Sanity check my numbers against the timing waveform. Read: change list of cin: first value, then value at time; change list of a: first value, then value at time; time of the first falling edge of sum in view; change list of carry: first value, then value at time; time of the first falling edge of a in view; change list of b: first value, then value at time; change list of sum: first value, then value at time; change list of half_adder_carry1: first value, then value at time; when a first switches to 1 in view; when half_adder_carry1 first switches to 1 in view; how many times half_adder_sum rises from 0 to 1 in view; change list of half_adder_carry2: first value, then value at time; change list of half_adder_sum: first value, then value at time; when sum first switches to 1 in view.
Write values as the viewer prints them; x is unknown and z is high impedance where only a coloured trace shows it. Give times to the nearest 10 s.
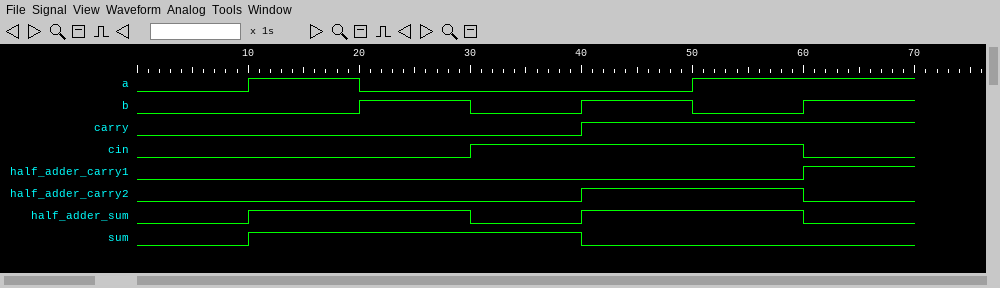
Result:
0, 1 at 30 s, 0 at 60 s
0, 1 at 10 s, 0 at 20 s, 1 at 50 s
40 s
0, 1 at 40 s
20 s
0, 1 at 20 s, 0 at 30 s, 1 at 40 s, 0 at 50 s, 1 at 60 s
0, 1 at 10 s, 0 at 40 s
0, 1 at 60 s
10 s
60 s
2
0, 1 at 40 s, 0 at 60 s
0, 1 at 10 s, 0 at 30 s, 1 at 40 s, 0 at 60 s
10 s
